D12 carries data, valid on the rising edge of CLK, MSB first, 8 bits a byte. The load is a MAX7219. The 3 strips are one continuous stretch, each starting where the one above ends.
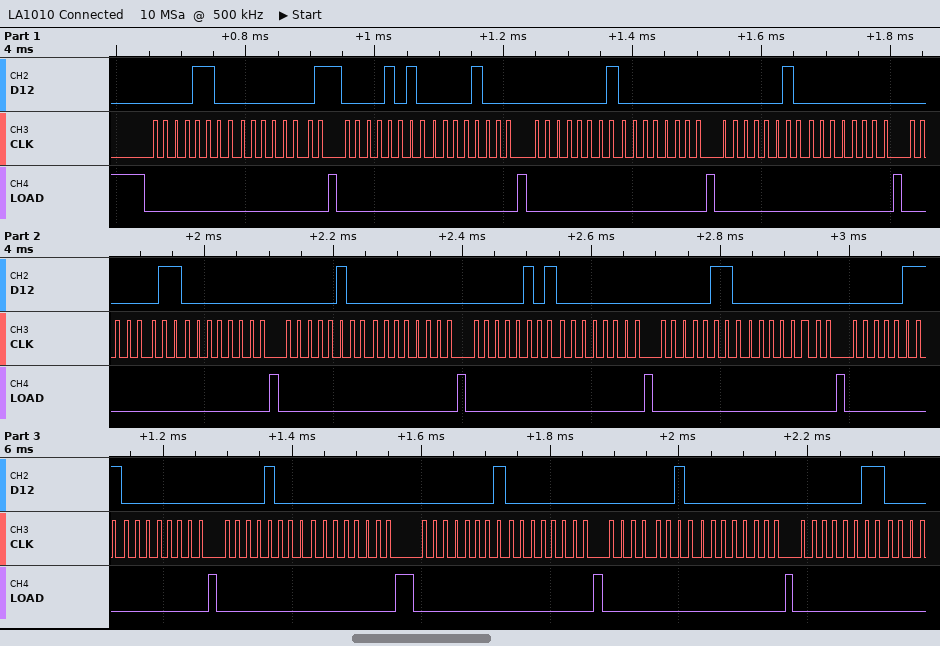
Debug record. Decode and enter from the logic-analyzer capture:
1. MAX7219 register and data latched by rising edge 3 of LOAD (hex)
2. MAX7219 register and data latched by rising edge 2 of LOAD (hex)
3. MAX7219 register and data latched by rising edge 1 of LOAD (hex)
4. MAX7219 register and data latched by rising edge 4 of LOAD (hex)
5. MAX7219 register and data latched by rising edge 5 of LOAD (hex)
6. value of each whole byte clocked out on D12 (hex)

register 0x1, data 0x00
register 0xA, data 0x08
register 0xC, data 0x01
register 0x2, data 0x00
register 0x3, data 0x00
0C 01 0A 08 01 00 02 00 03 00 04 00 05 00 06 00 07 00 08 00 01 00 02 00 03
